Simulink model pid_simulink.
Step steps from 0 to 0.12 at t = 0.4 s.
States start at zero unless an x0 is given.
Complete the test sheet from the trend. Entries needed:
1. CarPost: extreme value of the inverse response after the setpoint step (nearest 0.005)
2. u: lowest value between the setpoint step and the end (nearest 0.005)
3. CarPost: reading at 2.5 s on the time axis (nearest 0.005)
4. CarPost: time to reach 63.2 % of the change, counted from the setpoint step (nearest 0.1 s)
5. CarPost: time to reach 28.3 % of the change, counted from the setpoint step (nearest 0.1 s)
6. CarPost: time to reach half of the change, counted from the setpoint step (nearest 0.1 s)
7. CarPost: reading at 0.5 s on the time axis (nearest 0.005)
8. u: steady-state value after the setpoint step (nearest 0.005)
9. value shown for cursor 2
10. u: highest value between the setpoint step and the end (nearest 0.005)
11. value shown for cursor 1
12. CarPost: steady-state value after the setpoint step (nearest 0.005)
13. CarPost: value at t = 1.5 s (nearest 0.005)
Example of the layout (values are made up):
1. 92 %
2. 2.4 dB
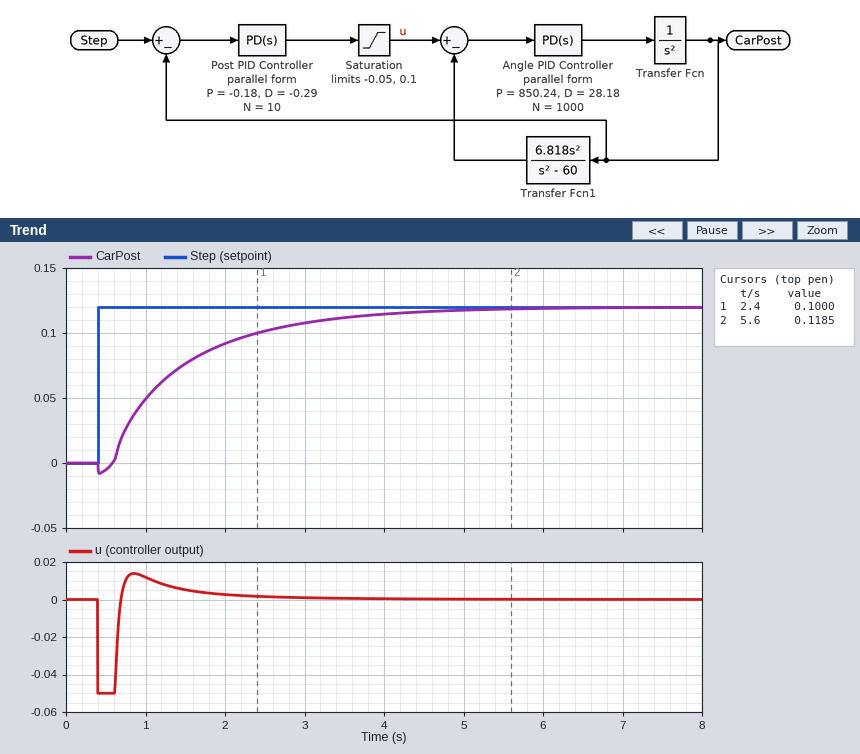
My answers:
1. -0.010
2. -0.050
3. 0.100
4. 1.1 s
5. 0.4 s
6. 0.8 s
7. -0.005
8. 0.000
9. 0.1185
10. 0.015
11. 0.1000
12. 0.120
13. 0.075
